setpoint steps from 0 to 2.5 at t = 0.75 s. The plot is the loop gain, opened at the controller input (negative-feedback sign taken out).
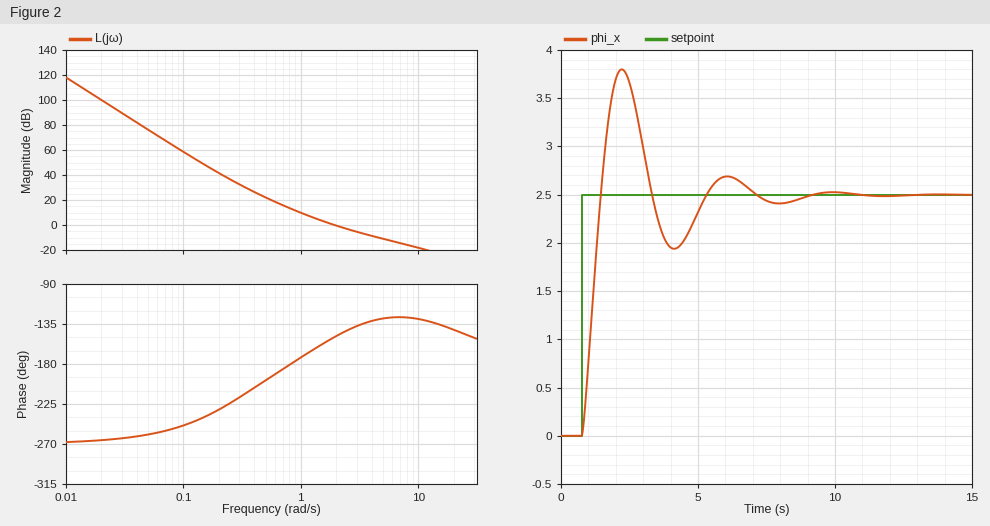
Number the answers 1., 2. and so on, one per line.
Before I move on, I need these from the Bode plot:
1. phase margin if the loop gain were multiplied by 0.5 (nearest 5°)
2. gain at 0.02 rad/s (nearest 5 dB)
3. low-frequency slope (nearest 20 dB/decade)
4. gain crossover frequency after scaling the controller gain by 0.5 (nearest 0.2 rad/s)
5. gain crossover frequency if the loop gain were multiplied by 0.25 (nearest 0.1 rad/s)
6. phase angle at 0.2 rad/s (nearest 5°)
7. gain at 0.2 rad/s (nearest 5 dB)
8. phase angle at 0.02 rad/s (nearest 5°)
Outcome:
1. 15°
2. 100 dB
3. -60 dB/decade
4. 1.2 rad/s
5. 0.9 rad/s
6. -230°
7. 40 dB
8. -265°
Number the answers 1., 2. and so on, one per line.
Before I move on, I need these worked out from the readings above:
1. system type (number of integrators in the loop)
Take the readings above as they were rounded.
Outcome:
1. 3
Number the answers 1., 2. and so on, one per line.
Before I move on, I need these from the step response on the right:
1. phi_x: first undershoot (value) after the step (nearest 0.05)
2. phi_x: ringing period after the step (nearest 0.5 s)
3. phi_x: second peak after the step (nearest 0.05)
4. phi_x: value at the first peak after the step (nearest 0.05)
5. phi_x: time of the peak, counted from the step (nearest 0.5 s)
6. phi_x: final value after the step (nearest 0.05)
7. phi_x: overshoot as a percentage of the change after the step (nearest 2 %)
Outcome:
1. 1.95
2. 4.0 s
3. 2.70
4. 3.80
5. 1.5 s
6. 2.50
7. 52 %
